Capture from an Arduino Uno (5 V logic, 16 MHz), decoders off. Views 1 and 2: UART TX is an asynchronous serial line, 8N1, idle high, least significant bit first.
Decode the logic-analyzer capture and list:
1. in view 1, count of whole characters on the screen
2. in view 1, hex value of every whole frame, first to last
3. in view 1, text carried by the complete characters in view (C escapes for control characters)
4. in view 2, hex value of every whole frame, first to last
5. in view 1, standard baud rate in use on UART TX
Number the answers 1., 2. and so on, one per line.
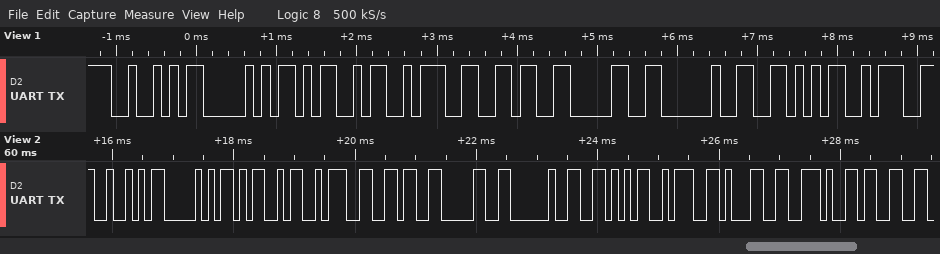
1. 9
2. 0x52 0x50 0x4D 0x3A 0x36 0x30 0x20 0x56 0x3A
3. "RPM:60 V:"
4. 52 50 4D 3A 36 30 20 56 3A 31 2E 33
5. 9600 baud
